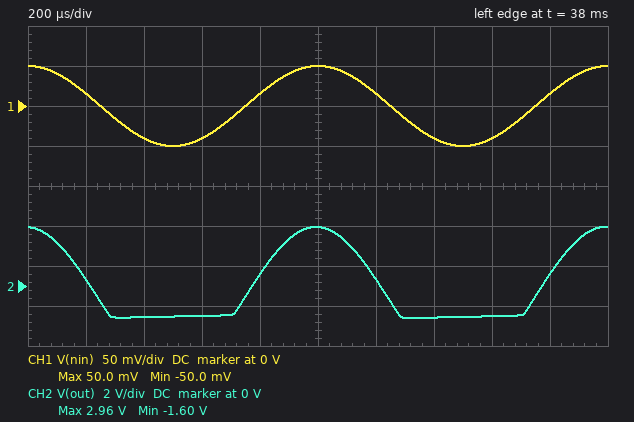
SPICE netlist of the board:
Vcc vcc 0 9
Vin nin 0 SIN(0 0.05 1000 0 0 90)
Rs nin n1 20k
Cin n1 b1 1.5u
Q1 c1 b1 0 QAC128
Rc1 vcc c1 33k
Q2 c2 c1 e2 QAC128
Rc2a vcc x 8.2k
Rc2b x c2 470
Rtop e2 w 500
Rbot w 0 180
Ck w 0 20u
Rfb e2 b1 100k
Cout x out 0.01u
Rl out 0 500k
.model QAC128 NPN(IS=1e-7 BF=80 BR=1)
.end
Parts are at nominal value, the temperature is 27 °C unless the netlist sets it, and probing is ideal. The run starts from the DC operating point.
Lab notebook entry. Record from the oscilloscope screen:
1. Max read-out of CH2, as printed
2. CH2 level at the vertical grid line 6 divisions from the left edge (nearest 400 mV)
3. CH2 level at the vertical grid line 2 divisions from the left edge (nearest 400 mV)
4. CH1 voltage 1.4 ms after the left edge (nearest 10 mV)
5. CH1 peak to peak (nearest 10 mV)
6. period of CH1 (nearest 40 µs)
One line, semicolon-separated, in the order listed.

2.96 V; 400 mV; -1.6 V; -40 mV; 100 mV; 1.00 ms
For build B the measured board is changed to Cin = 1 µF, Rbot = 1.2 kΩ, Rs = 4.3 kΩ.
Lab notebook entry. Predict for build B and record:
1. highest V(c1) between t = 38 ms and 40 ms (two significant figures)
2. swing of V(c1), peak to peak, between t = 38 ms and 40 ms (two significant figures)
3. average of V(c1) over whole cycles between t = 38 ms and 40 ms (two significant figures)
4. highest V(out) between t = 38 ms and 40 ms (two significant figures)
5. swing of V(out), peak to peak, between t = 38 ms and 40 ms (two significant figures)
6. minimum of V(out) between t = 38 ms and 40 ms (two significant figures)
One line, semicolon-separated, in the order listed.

1.3 V; 1.2 V; 670 mV; 3.5 V; 7.7 V; -4.2 V
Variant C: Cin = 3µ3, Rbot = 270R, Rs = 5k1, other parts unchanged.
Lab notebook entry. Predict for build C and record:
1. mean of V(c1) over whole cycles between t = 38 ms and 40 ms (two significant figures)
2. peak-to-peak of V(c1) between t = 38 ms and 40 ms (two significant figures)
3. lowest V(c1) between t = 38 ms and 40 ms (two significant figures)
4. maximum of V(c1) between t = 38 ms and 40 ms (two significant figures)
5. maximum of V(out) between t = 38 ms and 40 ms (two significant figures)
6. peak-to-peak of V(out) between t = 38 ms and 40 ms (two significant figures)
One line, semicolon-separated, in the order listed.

720 mV; 880 mV; 130 mV; 1.0 V; 5.3 V; 7.9 V
